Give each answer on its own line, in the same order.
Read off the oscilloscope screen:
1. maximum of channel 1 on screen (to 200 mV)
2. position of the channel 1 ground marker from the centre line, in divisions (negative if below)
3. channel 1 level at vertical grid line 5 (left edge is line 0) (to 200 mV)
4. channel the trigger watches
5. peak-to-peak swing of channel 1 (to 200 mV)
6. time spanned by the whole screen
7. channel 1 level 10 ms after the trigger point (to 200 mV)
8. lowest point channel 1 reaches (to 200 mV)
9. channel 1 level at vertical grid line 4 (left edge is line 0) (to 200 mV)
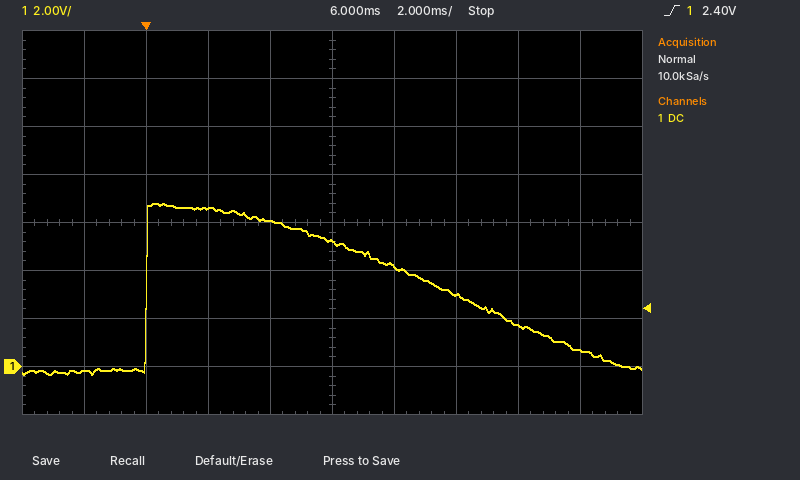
6.8 V
-3.0 div
5.2 V
channel 1
7.2 V
20 ms
3.0 V
-400 mV
6.0 V
